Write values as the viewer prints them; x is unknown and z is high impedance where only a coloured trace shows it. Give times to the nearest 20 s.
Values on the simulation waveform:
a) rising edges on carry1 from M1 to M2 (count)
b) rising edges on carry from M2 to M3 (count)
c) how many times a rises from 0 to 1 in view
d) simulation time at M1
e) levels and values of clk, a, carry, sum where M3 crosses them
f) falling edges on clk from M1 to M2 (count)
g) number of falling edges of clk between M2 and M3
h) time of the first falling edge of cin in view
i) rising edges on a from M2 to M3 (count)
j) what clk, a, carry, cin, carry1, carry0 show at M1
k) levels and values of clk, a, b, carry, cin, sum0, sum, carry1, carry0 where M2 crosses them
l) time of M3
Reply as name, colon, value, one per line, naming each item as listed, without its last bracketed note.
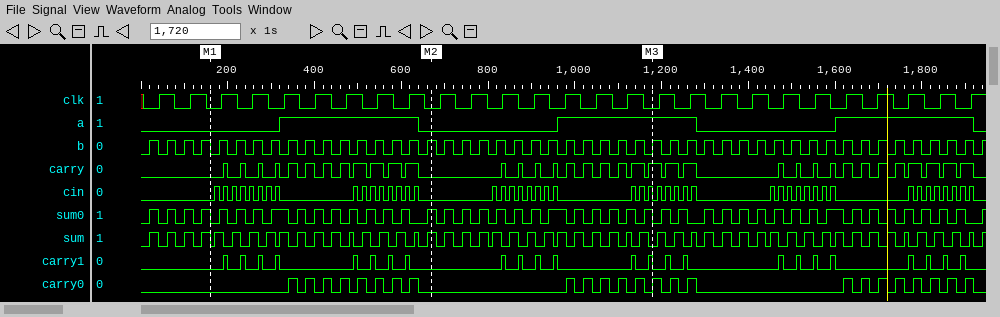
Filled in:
rising edges on carry1 from M1 to M2: 8
rising edges on carry from M2 to M3: 10
how many times a rises from 0 to 1 in view: 3
simulation time at M1: 160 s
levels and values of clk, a, carry, sum where M3 crosses them: clk=0, a=1, carry=1, sum=0
falling edges on clk from M1 to M2: 7
number of falling edges of clk between M2 and M3: 7
time of the first falling edge of cin in view: 180 s
rising edges on a from M2 to M3: 1
what clk, a, carry, cin, carry1, carry0 show at M1: clk=0, a=0, carry=0, cin=0, carry1=0, carry0=0
levels and values of clk, a, b, carry, cin, sum0, sum, carry1, carry0 where M2 crosses them: clk=0, a=0, b=1, carry=0, cin=0, sum0=1, sum=1, carry1=0, carry0=0
time of M3: 1180 s
